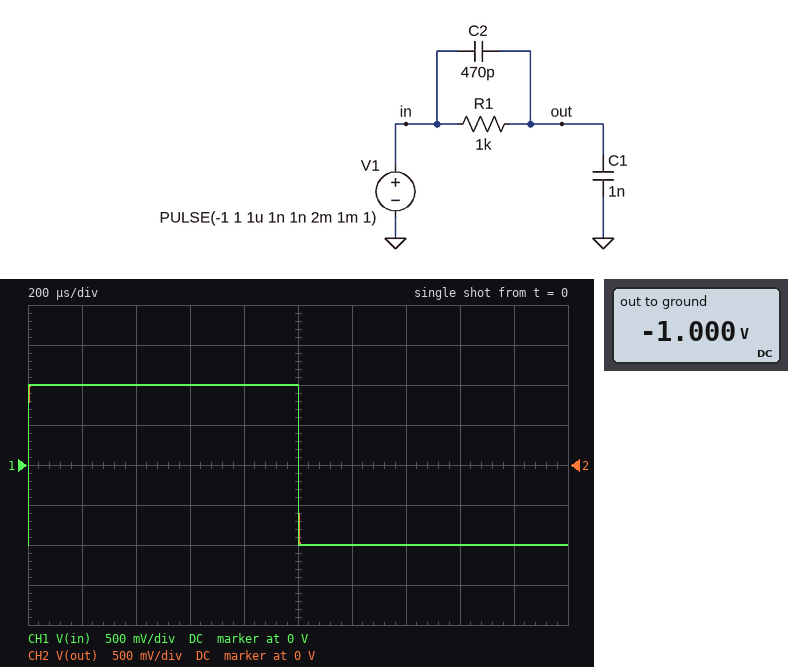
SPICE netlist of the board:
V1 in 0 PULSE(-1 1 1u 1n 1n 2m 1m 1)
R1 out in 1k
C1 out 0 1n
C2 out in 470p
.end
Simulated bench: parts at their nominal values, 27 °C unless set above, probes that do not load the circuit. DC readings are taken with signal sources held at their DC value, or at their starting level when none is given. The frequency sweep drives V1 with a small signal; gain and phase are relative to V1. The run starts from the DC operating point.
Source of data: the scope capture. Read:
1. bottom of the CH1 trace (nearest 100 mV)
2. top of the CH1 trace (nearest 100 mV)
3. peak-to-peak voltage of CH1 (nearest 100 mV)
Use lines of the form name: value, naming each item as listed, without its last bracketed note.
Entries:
bottom of the CH1 trace: -1.0 V
top of the CH1 trace: 1.0 V
peak-to-peak voltage of CH1: 2.0 V
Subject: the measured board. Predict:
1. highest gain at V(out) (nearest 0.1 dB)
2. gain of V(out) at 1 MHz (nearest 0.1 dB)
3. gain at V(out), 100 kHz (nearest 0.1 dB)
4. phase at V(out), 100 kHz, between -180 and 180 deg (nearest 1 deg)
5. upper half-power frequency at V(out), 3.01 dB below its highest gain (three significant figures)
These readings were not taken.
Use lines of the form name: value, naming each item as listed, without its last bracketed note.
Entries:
highest gain at V(out): 0 dB
gain of V(out) at 1 MHz: -9.5 dB
gain at V(out), 100 kHz: -2.3 dB
phase at V(out), 100 kHz, between -180 and 180 deg: -26 deg
upper half-power frequency at V(out), 3.01 dB below its highest gain: 121 kHz
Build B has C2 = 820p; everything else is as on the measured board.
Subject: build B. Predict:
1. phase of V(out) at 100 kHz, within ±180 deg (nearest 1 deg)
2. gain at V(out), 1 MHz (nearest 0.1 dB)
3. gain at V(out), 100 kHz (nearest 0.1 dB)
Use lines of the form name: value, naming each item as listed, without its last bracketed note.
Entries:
phase of V(out) at 100 kHz, within ±180 deg: -22 deg
gain at V(out), 1 MHz: -6.8 dB
gain at V(out), 100 kHz: -2.6 dB
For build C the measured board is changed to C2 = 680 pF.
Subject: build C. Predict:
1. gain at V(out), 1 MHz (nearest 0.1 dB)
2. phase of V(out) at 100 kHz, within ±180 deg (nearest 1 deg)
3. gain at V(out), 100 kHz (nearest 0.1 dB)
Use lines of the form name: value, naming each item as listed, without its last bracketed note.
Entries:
gain at V(out), 1 MHz: -7.7 dB
phase of V(out) at 100 kHz, within ±180 deg: -23 deg
gain at V(out), 100 kHz: -2.5 dB
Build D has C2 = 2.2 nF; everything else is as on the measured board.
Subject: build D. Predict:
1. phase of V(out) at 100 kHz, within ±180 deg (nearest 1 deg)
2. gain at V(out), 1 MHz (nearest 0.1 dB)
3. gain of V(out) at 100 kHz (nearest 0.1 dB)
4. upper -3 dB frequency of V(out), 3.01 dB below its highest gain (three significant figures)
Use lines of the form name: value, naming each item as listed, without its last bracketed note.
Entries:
phase of V(out) at 100 kHz, within ±180 deg: -9 deg
gain at V(out), 1 MHz: -3.2 dB
gain of V(out) at 100 kHz: -2.4 dB
upper -3 dB frequency of V(out), 3.01 dB below its highest gain: 213 kHz
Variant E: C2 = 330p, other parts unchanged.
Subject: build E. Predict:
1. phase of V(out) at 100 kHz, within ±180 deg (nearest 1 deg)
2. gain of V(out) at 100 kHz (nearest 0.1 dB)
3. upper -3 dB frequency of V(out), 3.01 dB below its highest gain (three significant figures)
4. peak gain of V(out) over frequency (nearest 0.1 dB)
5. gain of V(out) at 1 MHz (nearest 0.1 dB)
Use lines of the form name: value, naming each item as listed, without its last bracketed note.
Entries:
phase of V(out) at 100 kHz, within ±180 deg: -28 deg
gain of V(out) at 100 kHz: -2.1 dB
upper -3 dB frequency of V(out), 3.01 dB below its highest gain: 128 kHz
peak gain of V(out) over frequency: 0 dB
gain of V(out) at 1 MHz: -11.3 dB
